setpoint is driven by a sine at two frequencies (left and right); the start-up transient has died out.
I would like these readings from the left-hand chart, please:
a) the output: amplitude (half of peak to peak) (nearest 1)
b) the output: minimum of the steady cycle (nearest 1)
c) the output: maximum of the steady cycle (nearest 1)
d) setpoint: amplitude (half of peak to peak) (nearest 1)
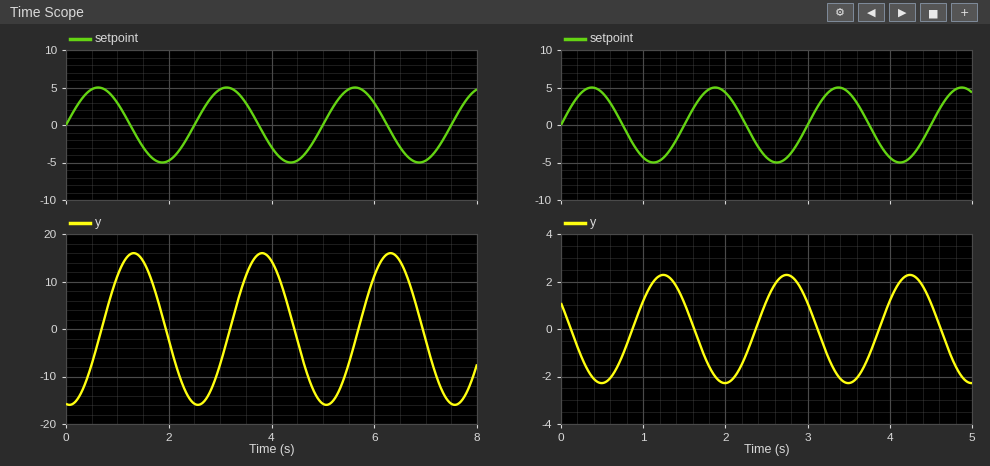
16
-16
16
5
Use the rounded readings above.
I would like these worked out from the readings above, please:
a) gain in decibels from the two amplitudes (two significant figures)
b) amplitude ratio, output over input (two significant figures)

10 dB
3.2
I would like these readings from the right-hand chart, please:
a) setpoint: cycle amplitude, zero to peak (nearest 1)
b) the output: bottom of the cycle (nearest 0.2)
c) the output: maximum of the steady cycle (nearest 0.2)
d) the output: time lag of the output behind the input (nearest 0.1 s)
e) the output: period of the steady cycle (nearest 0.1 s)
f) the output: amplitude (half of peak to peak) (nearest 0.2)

5
-2.2
2.2
0.9 s
1.5 s
2.2
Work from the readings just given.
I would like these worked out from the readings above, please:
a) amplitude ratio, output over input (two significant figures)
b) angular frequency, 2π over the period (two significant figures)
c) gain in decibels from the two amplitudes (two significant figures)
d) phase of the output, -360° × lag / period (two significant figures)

0.44
4.2 rad/s
-7.1 dB
-220°
